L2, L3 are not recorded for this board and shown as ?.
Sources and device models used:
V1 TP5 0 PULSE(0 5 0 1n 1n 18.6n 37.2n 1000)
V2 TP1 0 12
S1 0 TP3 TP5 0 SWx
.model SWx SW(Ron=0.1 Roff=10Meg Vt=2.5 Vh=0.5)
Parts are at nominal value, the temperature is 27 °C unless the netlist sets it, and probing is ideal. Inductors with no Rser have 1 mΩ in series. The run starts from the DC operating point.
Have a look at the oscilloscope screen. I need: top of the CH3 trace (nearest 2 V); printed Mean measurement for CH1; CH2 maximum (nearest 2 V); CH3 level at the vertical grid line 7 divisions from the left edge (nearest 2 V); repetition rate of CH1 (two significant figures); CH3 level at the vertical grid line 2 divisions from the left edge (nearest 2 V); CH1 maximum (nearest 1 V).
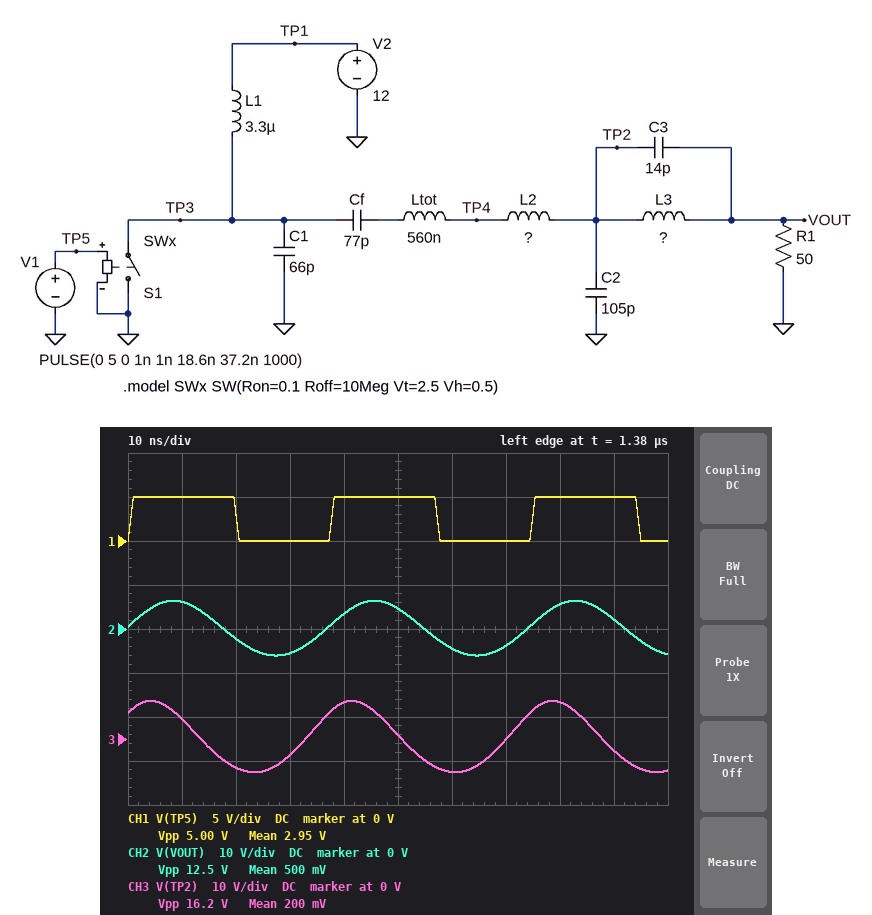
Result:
8 V
2.95 V
6 V
0 V
27 MHz
-6 V
5 V
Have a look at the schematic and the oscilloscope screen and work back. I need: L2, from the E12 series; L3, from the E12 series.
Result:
1 µH
220 nH
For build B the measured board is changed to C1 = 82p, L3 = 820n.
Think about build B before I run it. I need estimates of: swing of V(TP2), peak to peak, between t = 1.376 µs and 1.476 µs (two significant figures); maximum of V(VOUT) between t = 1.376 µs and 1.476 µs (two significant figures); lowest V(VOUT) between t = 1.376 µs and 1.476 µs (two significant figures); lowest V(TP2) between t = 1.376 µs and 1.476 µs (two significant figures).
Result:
25 V
3.0 V
-2.9 V
-13 V
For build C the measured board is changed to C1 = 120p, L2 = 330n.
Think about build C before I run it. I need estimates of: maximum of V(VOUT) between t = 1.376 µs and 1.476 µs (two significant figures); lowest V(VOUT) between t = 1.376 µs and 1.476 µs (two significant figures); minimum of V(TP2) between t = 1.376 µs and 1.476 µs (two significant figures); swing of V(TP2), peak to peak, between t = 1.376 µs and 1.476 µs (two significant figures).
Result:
15 V
-14 V
-18 V
37 V
